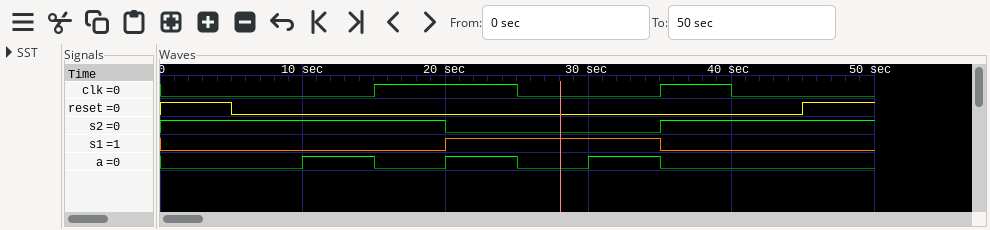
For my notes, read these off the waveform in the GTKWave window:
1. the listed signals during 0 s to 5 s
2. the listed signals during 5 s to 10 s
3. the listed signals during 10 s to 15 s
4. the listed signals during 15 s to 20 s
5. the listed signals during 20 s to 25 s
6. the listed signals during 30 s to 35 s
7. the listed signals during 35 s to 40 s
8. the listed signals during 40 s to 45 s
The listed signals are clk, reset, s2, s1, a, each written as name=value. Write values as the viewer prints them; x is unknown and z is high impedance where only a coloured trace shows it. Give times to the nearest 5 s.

clk=0, reset=1, s2=1, s1=0, a=0
clk=0, reset=0, s2=1, s1=0, a=0
clk=0, reset=0, s2=1, s1=0, a=1
clk=1, reset=0, s2=1, s1=0, a=0
clk=1, reset=0, s2=0, s1=1, a=1
clk=0, reset=0, s2=0, s1=1, a=1
clk=1, reset=0, s2=1, s1=0, a=0
clk=0, reset=0, s2=1, s1=0, a=0
